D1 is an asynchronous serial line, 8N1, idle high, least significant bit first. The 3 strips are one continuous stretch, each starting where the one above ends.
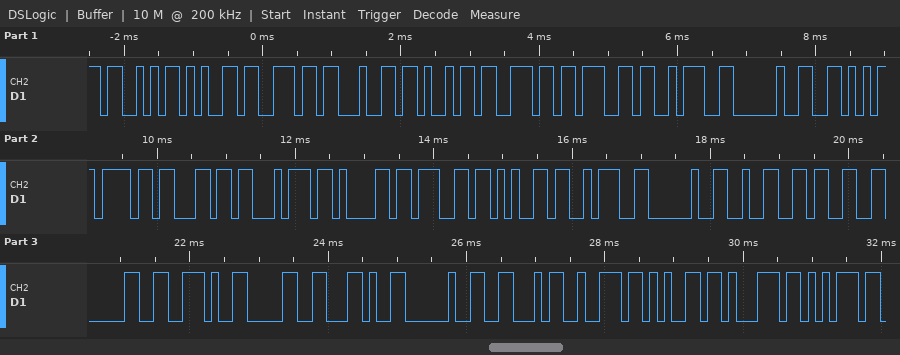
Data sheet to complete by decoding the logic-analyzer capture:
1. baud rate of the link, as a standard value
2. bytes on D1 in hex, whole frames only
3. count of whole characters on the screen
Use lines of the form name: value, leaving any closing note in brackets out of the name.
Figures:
baud rate of the link, as a standard value: 9600 baud
bytes on D1 in hex, whole frames only: 53 65 6E 64 69 6E 67 3A 20 56 6F 6C 74 61 67 65 3A 20 32 33 30 2E 30 2C 20 46 72 65 71 75
count of whole characters on the screen: 30
